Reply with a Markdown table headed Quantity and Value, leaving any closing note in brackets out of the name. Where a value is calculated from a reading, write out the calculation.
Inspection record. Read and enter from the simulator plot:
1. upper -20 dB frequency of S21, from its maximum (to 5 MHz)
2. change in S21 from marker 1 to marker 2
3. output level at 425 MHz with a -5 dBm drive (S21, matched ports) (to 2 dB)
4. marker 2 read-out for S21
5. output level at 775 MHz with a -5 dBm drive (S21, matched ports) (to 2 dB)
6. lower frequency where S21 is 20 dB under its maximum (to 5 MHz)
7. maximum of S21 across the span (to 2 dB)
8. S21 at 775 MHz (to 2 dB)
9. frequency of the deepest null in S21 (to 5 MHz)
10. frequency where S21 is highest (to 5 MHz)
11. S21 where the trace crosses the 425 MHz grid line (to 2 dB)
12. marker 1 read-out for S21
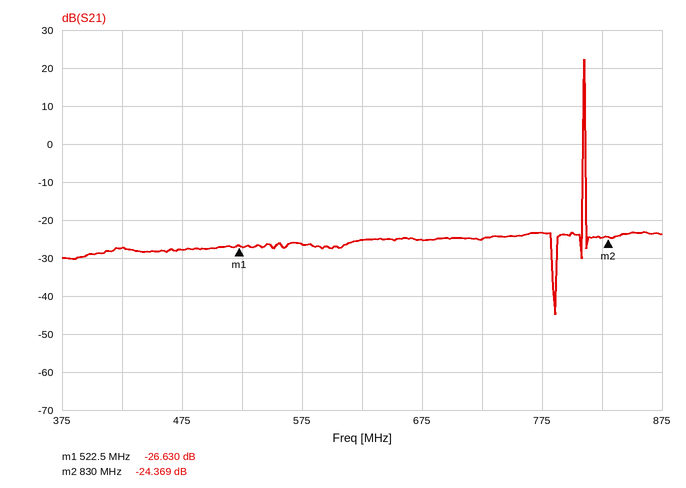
| Quantity | Value |
|---|---|
| upper -20 dB frequency of S21, from its maximum | 810 MHz |
| change in S21 from marker 1 to marker 2 | -24.369 − (-26.63) = 2.261 dB |
| output level at 425 MHz with a -5 dBm drive (S21, matched ports) | -5 dBm + (-28 dB) = -32 dBm |
| marker 2 read-out for S21 | -24.369 dB |
| output level at 775 MHz with a -5 dBm drive (S21, matched ports) | -5 dBm + (-24 dB) = -28 dBm |
| lower frequency where S21 is 20 dB under its maximum | 810 MHz |
| maximum of S21 across the span | 22 dB |
| S21 at 775 MHz | -24 dB |
| frequency of the deepest null in S21 | 785 MHz |
| frequency where S21 is highest | 810 MHz |
| S21 where the trace crosses the 425 MHz grid line | -28 dB |
| marker 1 read-out for S21 | -26.630 dB |
